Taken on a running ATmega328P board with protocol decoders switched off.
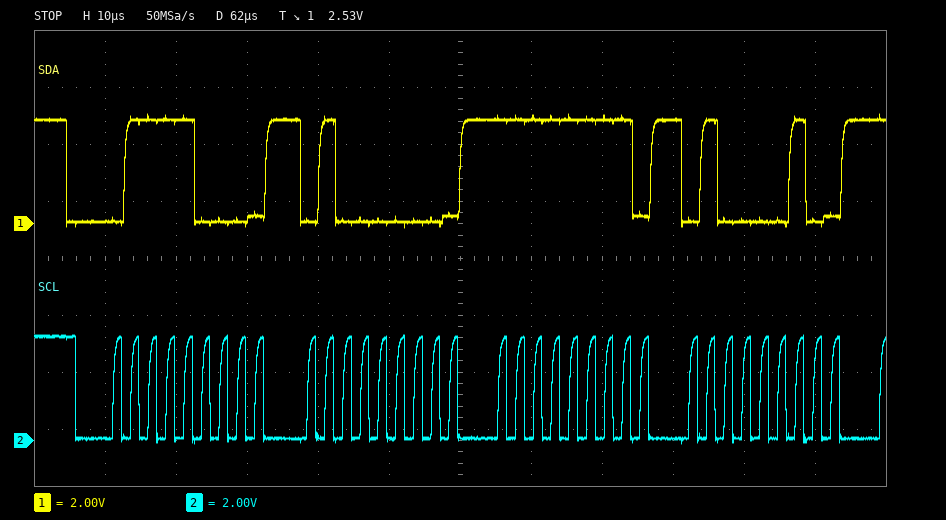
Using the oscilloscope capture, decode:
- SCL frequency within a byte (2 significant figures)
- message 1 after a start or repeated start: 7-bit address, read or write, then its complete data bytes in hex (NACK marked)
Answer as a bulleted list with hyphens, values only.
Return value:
- 400 kHz
- 0x3C write: 40 FF 42
